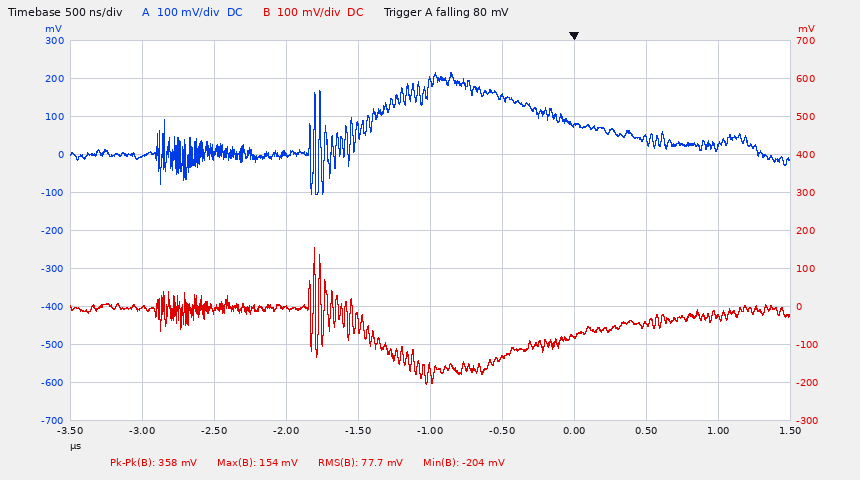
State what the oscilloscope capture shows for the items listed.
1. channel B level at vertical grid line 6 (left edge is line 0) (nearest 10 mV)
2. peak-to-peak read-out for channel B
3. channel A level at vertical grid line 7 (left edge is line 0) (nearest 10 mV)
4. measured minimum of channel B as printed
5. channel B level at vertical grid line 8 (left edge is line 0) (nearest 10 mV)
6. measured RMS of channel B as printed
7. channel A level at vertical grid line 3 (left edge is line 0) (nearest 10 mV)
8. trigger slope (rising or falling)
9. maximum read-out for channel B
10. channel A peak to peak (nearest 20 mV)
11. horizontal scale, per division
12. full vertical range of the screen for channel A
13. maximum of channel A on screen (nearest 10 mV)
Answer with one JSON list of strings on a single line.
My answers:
["-140 mV", "358 mV", "80 mV", "-204 mV", "-50 mV", "77.7 mV", "0 mV", "falling", "154 mV", "320 mV", "500 ns", "1 V", "220 mV"]
